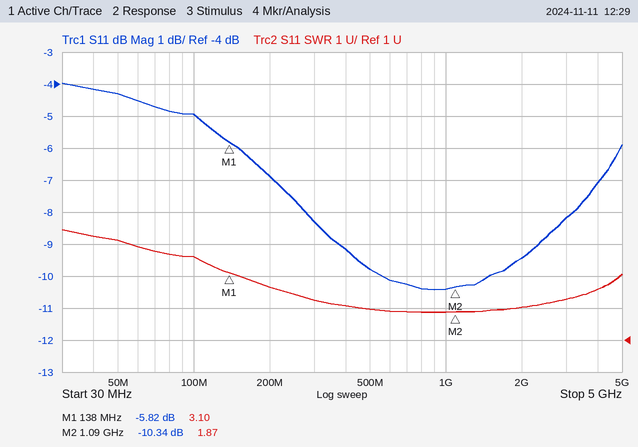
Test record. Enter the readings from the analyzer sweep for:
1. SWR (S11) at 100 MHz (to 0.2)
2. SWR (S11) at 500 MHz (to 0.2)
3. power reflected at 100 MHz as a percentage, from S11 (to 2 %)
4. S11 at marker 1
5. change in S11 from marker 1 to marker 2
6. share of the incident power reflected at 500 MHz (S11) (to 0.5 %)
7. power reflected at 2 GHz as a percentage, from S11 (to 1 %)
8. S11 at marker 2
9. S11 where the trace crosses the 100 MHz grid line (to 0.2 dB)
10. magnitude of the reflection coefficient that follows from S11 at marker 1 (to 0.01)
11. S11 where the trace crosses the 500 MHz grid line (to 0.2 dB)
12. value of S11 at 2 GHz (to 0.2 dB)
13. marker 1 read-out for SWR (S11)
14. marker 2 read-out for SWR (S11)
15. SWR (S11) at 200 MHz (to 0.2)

3.6
2.0
32 %
-5.82 dB
-4.52 dB
10.5 %
11 %
-10.34 dB
-5.0 dB
0.51
-9.8 dB
-9.4 dB
3.10
1.87
2.6
